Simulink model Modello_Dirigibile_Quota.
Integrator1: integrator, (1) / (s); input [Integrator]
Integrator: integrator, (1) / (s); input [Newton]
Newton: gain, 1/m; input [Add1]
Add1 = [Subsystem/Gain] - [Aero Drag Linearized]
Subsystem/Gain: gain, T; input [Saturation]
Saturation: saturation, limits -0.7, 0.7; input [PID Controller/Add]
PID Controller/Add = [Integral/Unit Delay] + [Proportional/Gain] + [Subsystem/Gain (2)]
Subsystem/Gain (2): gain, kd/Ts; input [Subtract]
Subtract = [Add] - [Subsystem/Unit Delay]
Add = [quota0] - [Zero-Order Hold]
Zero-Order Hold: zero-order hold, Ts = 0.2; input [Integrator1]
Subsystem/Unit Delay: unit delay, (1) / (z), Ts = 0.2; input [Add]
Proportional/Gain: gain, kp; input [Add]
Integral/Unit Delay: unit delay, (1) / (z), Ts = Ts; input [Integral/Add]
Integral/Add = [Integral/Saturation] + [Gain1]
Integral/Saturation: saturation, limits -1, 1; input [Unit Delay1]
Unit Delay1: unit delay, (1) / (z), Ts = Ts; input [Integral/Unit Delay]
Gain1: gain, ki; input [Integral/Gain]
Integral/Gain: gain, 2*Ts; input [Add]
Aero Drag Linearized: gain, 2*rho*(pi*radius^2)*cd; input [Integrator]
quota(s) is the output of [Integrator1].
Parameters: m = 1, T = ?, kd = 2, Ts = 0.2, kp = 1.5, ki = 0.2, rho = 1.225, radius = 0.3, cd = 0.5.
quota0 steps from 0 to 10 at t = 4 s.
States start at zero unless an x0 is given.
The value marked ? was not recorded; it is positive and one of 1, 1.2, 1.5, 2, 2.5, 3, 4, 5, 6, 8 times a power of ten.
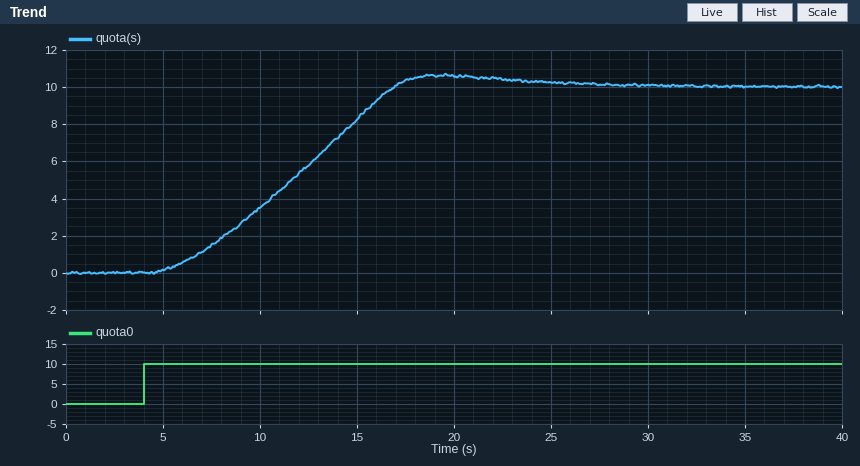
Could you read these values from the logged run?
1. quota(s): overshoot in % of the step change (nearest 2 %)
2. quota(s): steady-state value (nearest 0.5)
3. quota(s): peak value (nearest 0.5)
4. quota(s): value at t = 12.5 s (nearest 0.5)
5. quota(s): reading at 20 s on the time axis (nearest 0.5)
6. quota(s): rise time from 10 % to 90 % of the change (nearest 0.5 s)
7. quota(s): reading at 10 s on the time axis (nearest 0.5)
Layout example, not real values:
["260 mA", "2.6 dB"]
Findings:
["6 %", "10.0", "10.5", "6.0", "10.5", "9.0 s", "3.5"]
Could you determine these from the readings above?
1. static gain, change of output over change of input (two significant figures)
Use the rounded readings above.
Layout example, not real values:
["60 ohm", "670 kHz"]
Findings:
["1.0"]
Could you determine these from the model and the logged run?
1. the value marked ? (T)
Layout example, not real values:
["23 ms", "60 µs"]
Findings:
["0.5"]
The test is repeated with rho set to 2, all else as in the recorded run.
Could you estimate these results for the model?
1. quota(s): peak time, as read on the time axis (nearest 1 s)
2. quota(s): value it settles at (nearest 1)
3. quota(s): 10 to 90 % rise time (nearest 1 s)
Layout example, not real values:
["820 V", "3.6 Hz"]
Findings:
["25 s", "10", "13 s"]
